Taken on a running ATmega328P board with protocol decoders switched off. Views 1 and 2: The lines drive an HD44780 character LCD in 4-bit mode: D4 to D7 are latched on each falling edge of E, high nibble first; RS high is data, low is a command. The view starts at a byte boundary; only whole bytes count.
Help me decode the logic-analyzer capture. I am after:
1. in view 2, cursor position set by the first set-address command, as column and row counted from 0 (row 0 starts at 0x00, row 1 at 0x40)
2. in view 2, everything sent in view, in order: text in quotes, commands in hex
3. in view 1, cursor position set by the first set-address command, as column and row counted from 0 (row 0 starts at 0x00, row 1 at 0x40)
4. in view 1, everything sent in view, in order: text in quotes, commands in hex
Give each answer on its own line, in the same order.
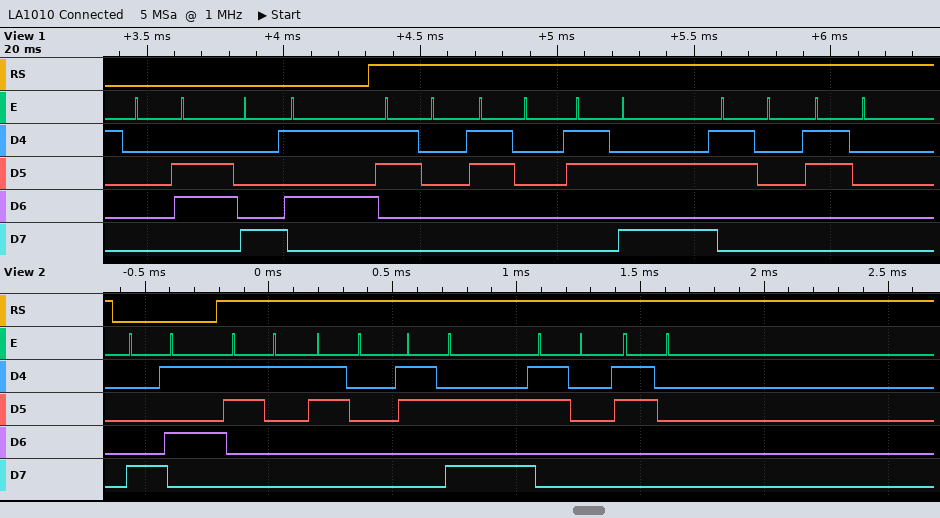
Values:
column 5, row 0
0x85 "10:00"
column 5, row 0
0x06 0x85 "00:00"
